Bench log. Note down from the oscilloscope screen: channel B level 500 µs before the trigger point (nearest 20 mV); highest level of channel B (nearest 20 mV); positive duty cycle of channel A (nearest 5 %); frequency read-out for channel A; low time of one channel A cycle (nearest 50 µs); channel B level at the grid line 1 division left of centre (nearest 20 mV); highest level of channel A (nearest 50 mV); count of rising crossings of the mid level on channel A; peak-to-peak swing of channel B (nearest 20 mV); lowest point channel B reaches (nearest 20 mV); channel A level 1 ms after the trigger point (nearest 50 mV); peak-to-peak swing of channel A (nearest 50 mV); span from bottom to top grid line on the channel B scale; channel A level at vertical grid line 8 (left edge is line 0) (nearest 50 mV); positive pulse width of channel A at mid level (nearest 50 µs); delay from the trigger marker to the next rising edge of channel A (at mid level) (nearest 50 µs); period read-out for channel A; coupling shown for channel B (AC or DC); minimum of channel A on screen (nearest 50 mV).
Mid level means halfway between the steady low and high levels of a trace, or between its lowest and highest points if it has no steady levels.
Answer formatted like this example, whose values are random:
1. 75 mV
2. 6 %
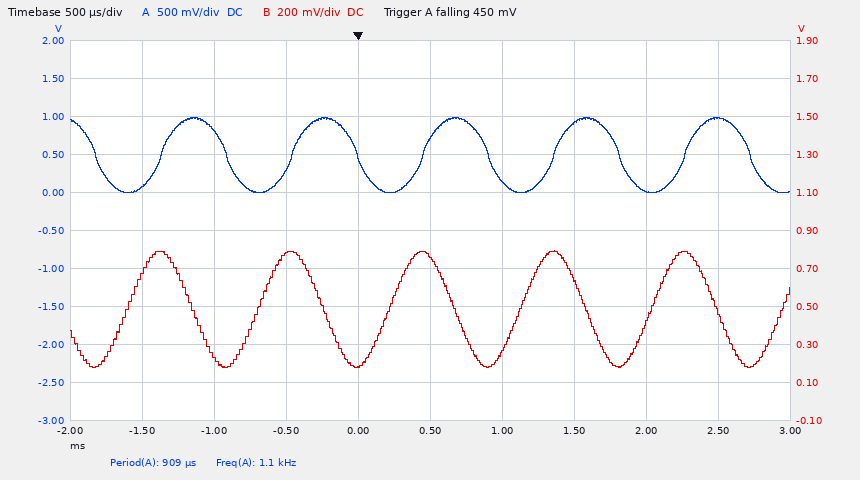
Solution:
1. 780 mV
2. 800 mV
3. 50 %
4. 1.1 kHz
5. 450 µs
6. 180 mV
7. 1.00 V
8. 5
9. 620 mV
10. 180 mV
11. 150 mV
12. 1.00 V
13. 2 V
14. 0 mV
15. 450 µs
16. 450 µs
17. 909 µs
18. DC
19. 0 mV
